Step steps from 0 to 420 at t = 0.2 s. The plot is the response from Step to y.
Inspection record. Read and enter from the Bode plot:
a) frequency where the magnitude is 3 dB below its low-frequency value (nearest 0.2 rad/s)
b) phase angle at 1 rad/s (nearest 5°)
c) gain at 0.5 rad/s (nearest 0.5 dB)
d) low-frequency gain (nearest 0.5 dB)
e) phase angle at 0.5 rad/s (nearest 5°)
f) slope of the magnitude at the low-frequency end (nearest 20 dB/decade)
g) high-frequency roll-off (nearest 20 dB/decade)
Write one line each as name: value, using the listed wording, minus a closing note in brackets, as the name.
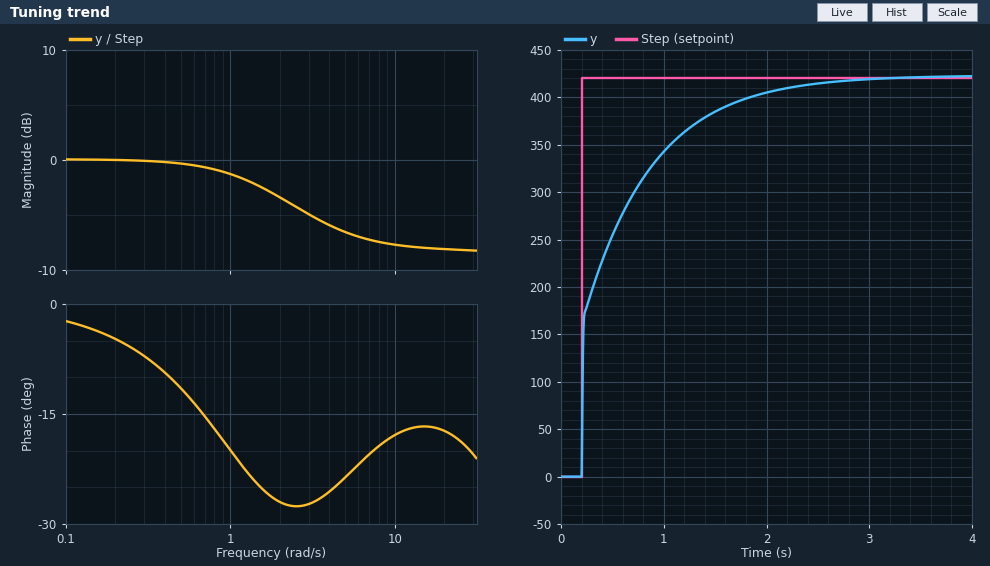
frequency where the magnitude is 3 dB below its low-frequency value: 1.8 rad/s
phase angle at 1 rad/s: -20°
gain at 0.5 rad/s: -0.5 dB
low-frequency gain: 0.0 dB
phase angle at 0.5 rad/s: -10°
slope of the magnitude at the low-frequency end: 0 dB/decade
high-frequency roll-off: 0 dB/decade
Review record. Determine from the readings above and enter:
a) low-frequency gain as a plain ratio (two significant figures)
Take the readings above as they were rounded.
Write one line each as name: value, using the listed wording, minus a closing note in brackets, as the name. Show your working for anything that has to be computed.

low-frequency gain as a plain ratio: 10^(0 / 20) = 1.0
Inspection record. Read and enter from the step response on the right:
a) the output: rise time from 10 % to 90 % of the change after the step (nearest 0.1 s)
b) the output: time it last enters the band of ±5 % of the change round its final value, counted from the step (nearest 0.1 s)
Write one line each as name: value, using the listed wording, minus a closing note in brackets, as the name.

the output: rise time from 10 % to 90 % of the change after the step: 1.2 s
the output: time it last enters the band of ±5 % of the change round its final value, counted from the step: 1.7 s
